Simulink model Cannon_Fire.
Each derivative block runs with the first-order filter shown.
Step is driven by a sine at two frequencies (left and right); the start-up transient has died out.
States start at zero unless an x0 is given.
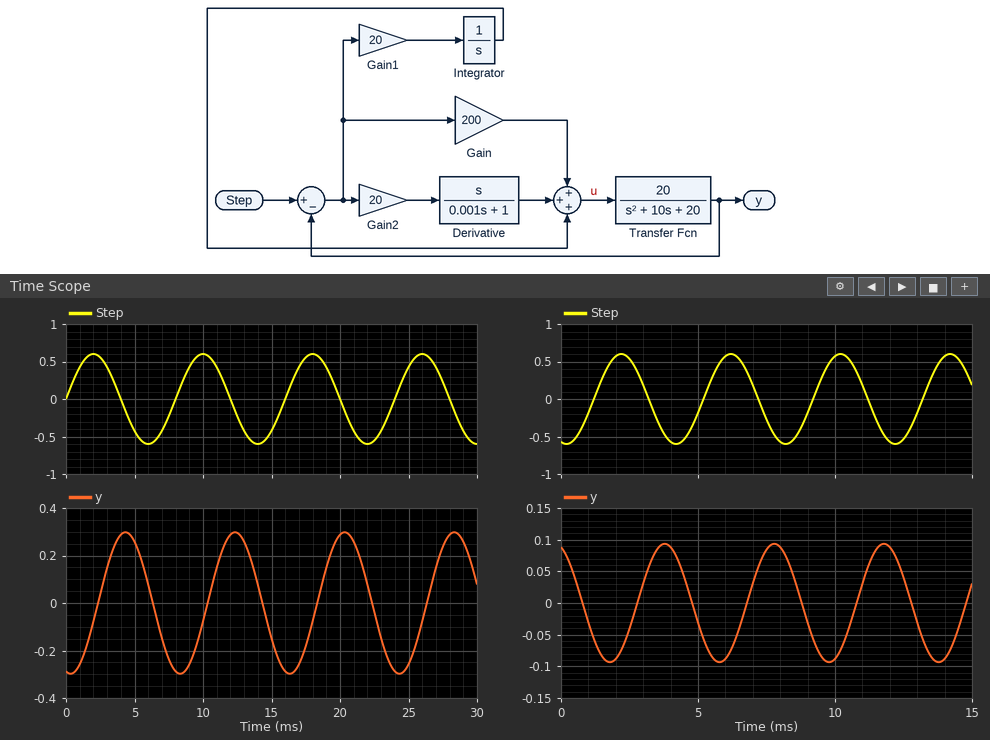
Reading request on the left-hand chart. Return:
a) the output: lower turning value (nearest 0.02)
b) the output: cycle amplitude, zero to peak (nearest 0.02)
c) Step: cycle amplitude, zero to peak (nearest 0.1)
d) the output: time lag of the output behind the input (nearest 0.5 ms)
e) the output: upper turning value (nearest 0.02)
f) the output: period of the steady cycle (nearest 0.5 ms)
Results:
-0.30
0.30
0.6
2.5 ms
0.30
8.0 ms
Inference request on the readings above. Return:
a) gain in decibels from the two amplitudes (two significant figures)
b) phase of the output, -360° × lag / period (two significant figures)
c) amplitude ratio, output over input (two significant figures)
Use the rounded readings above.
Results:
-6.0 dB
-110°
0.50
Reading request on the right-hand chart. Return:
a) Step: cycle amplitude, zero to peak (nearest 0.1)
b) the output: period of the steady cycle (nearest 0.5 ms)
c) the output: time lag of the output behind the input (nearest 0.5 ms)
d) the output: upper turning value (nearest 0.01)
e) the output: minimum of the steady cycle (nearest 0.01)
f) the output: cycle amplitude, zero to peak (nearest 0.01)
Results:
0.6
4.0 ms
1.5 ms
0.09
-0.09
0.09
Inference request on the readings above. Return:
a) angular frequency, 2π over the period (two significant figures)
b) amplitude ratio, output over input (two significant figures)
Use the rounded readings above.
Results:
1.6 rad/ms
0.15
